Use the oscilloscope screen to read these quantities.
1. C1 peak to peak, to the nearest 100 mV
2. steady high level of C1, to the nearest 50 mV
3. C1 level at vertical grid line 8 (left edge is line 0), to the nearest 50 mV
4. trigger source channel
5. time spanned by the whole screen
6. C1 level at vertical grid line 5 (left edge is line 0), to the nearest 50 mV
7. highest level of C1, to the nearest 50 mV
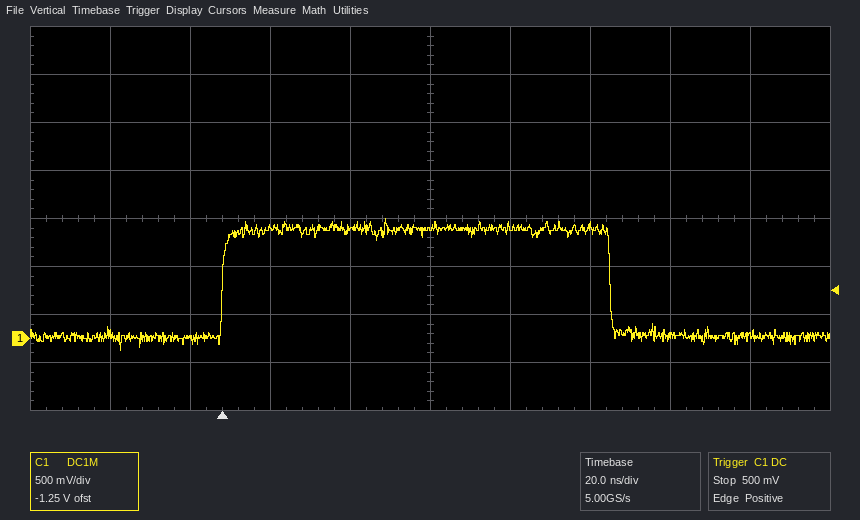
1.40 V
1.15 V
0 mV
C1
200 ns
1.15 V
1.25 V
